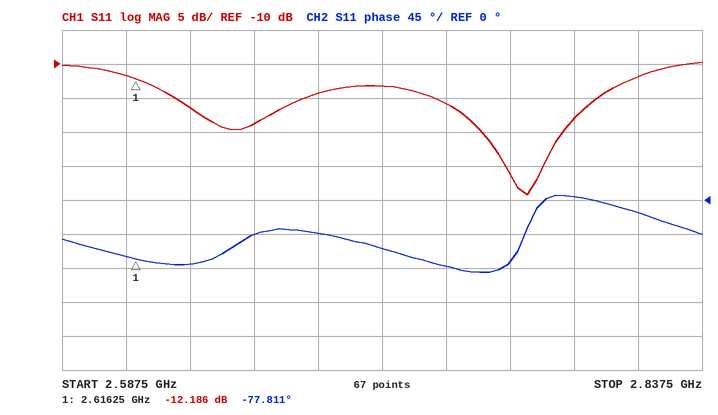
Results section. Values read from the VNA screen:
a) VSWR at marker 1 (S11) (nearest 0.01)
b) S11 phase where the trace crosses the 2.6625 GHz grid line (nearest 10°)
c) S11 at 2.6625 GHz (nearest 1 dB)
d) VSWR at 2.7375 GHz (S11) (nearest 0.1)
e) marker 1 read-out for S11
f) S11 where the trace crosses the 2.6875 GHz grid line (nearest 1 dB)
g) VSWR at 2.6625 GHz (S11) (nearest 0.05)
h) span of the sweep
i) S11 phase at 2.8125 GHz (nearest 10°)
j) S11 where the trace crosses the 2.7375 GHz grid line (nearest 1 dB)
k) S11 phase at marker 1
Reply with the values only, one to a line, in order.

1.65
-50°
-19 dB
1.4
-12.186 dB
-14 dB
1.25
250 MHz
-20°
-16 dB
-77.811°
